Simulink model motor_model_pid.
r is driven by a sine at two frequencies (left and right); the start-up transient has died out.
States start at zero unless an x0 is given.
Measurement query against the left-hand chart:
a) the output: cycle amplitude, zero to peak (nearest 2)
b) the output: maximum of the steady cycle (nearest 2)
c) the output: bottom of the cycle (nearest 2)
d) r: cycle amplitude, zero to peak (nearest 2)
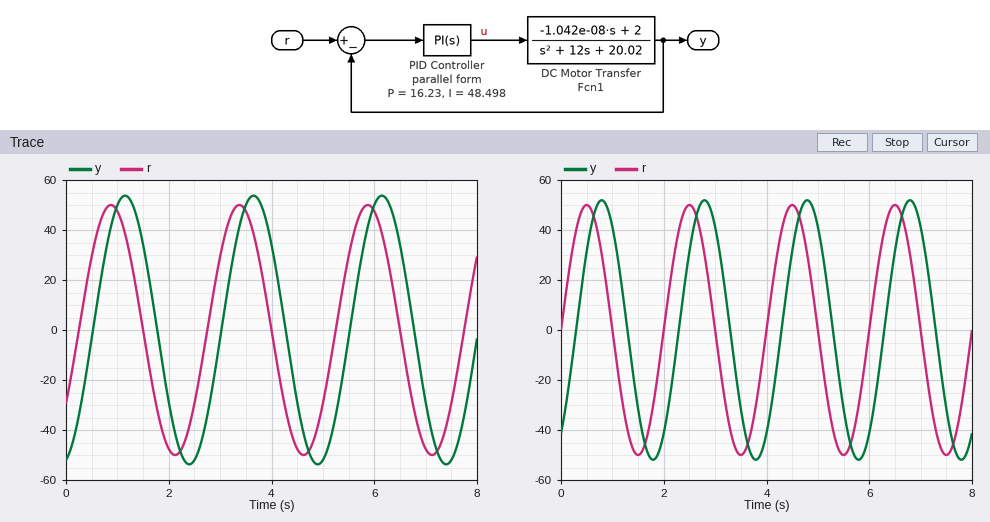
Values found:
54
54
-54
50
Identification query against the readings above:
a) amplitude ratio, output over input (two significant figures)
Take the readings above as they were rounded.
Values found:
1.1
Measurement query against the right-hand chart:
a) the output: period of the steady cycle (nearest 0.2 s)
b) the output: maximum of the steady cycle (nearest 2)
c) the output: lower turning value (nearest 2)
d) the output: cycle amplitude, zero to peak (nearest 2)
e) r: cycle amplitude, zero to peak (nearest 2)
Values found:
2.0 s
52
-52
52
50
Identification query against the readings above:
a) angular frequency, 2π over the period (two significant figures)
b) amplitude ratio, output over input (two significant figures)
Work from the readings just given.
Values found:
3.1 rad/s
1.0
